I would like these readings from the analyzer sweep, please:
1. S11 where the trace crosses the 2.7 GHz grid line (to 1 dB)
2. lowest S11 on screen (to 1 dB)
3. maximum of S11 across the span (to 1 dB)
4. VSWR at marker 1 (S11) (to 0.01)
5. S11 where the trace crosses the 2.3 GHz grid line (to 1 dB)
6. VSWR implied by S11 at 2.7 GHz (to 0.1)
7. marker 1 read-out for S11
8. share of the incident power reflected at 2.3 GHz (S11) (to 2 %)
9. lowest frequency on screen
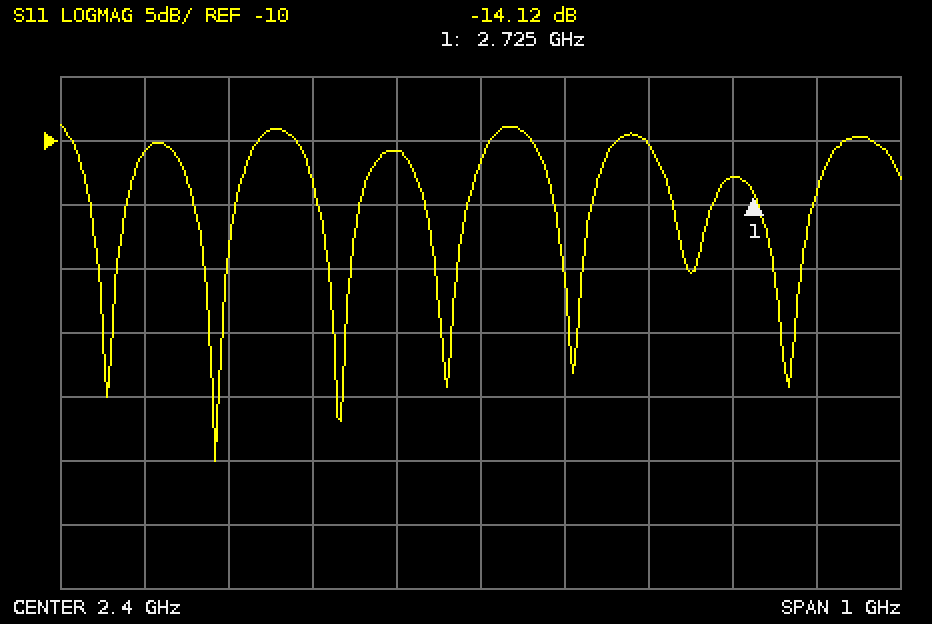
-13 dB
-35 dB
-9 dB
1.49
-11 dB
1.6
-14.12 dB
8 %
1.9 GHz
